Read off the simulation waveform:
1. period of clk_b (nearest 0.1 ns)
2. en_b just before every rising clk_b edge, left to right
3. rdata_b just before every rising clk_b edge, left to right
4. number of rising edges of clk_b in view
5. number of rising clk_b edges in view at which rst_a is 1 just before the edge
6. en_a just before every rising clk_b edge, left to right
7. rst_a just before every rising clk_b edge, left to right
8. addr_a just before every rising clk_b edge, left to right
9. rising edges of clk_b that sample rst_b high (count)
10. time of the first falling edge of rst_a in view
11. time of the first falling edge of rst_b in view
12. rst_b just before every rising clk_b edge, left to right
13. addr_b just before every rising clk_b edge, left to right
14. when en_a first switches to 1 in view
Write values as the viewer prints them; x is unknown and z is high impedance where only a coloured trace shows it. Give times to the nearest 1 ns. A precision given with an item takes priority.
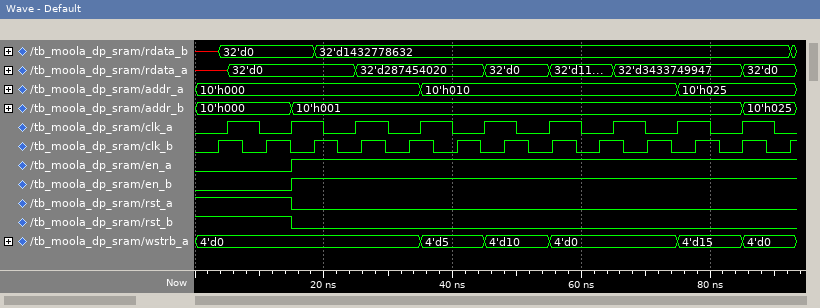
7.4 ns
0 0 1 1 1 1 1 1 1 1 1 1 1
x, 32'd0, 32'd0, 32'd1432778632, 32'd1432778632, 32'd1432778632, 32'd1432778632, 32'd1432778632, 32'd1432778632, 32'd1432778632, 32'd1432778632, 32'd1432778632, 32'd1432778632
13
2
0 0 1 1 1 1 1 1 1 1 1 1 1
1 1 0 0 0 0 0 0 0 0 0 0 0
10'h000, 10'h000, 10'h000, 10'h000, 10'h000, 10'h010, 10'h010, 10'h010, 10'h010, 10'h010, 10'h025, 10'h025, 10'h025
2
15 ns
15 ns
1 1 0 0 0 0 0 0 0 0 0 0 0
10'h000, 10'h000, 10'h001, 10'h001, 10'h001, 10'h001, 10'h001, 10'h001, 10'h001, 10'h001, 10'h001, 10'h001, 10'h025
15 ns
